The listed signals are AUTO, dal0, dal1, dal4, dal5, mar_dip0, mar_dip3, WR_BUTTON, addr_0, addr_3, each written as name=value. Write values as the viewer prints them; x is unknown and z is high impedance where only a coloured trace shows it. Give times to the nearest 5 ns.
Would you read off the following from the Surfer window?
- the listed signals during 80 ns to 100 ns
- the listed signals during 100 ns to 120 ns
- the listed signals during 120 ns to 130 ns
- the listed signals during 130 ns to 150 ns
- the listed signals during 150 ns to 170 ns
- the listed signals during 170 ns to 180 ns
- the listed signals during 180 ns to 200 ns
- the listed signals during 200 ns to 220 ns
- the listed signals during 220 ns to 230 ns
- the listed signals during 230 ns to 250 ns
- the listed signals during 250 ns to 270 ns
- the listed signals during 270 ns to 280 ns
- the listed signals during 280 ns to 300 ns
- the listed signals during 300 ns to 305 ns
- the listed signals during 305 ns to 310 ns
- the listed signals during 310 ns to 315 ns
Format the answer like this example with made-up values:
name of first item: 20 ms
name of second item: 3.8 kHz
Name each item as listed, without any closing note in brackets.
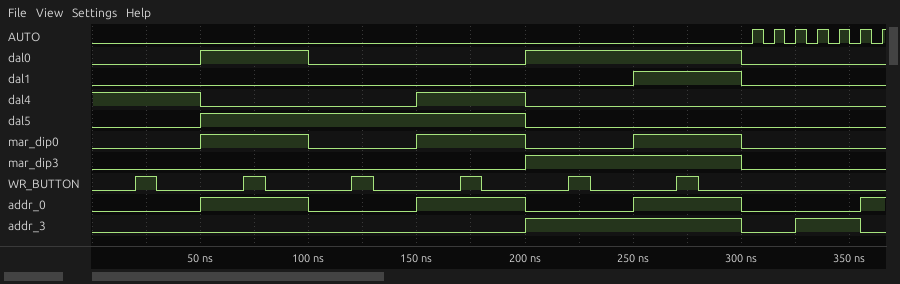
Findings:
the listed signals during 80 ns to 100 ns: AUTO=0, dal0=1, dal1=0, dal4=0, dal5=1, mar_dip0=1, mar_dip3=0, WR_BUTTON=0, addr_0=1, addr_3=0
the listed signals during 100 ns to 120 ns: AUTO=0, dal0=0, dal1=0, dal4=0, dal5=1, mar_dip0=0, mar_dip3=0, WR_BUTTON=0, addr_0=0, addr_3=0
the listed signals during 120 ns to 130 ns: AUTO=0, dal0=0, dal1=0, dal4=0, dal5=1, mar_dip0=0, mar_dip3=0, WR_BUTTON=1, addr_0=0, addr_3=0
the listed signals during 130 ns to 150 ns: AUTO=0, dal0=0, dal1=0, dal4=0, dal5=1, mar_dip0=0, mar_dip3=0, WR_BUTTON=0, addr_0=0, addr_3=0
the listed signals during 150 ns to 170 ns: AUTO=0, dal0=0, dal1=0, dal4=1, dal5=1, mar_dip0=1, mar_dip3=0, WR_BUTTON=0, addr_0=1, addr_3=0
the listed signals during 170 ns to 180 ns: AUTO=0, dal0=0, dal1=0, dal4=1, dal5=1, mar_dip0=1, mar_dip3=0, WR_BUTTON=1, addr_0=1, addr_3=0
the listed signals during 180 ns to 200 ns: AUTO=0, dal0=0, dal1=0, dal4=1, dal5=1, mar_dip0=1, mar_dip3=0, WR_BUTTON=0, addr_0=1, addr_3=0
the listed signals during 200 ns to 220 ns: AUTO=0, dal0=1, dal1=0, dal4=0, dal5=0, mar_dip0=0, mar_dip3=1, WR_BUTTON=0, addr_0=0, addr_3=1
the listed signals during 220 ns to 230 ns: AUTO=0, dal0=1, dal1=0, dal4=0, dal5=0, mar_dip0=0, mar_dip3=1, WR_BUTTON=1, addr_0=0, addr_3=1
the listed signals during 230 ns to 250 ns: AUTO=0, dal0=1, dal1=0, dal4=0, dal5=0, mar_dip0=0, mar_dip3=1, WR_BUTTON=0, addr_0=0, addr_3=1
the listed signals during 250 ns to 270 ns: AUTO=0, dal0=1, dal1=1, dal4=0, dal5=0, mar_dip0=1, mar_dip3=1, WR_BUTTON=0, addr_0=1, addr_3=1
the listed signals during 270 ns to 280 ns: AUTO=0, dal0=1, dal1=1, dal4=0, dal5=0, mar_dip0=1, mar_dip3=1, WR_BUTTON=1, addr_0=1, addr_3=1
the listed signals during 280 ns to 300 ns: AUTO=0, dal0=1, dal1=1, dal4=0, dal5=0, mar_dip0=1, mar_dip3=1, WR_BUTTON=0, addr_0=1, addr_3=1
the listed signals during 300 ns to 305 ns: AUTO=0, dal0=0, dal1=0, dal4=0, dal5=0, mar_dip0=0, mar_dip3=0, WR_BUTTON=0, addr_0=0, addr_3=0
the listed signals during 305 ns to 310 ns: AUTO=1, dal0=0, dal1=0, dal4=0, dal5=0, mar_dip0=0, mar_dip3=0, WR_BUTTON=0, addr_0=0, addr_3=0
the listed signals during 310 ns to 315 ns: AUTO=0, dal0=0, dal1=0, dal4=0, dal5=0, mar_dip0=0, mar_dip3=0, WR_BUTTON=0, addr_0=0, addr_3=0
